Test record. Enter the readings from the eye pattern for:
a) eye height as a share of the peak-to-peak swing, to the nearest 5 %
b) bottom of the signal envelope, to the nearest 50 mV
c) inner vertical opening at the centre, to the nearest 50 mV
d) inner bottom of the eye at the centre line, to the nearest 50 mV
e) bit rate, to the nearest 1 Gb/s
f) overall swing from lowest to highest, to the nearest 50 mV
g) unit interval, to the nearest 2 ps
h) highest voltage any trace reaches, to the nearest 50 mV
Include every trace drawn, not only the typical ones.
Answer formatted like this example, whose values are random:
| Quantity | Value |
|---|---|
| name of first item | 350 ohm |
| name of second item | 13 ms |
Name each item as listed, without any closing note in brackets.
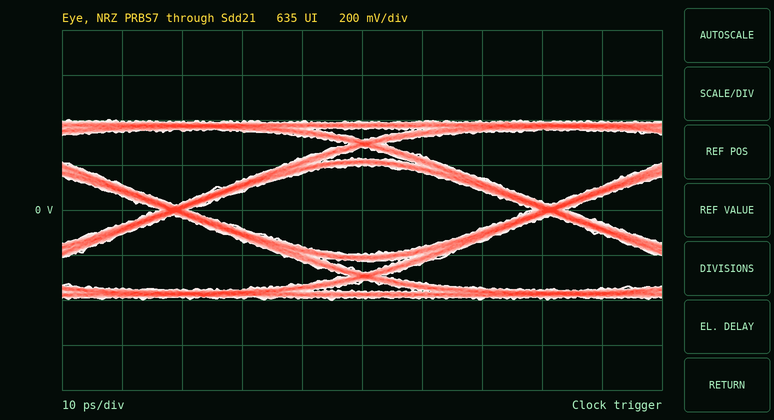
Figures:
| Quantity | Value |
|---|---|
| eye height as a share of the peak-to-peak swing, to the nearest 5 % | 50 % |
| bottom of the signal envelope, to the nearest 50 mV | -400 mV |
| inner vertical opening at the centre, to the nearest 50 mV | 400 mV |
| inner bottom of the eye at the centre line, to the nearest 50 mV | -200 mV |
| bit rate, to the nearest 1 Gb/s | 16 Gb/s |
| overall swing from lowest to highest, to the nearest 50 mV | 800 mV |
| unit interval, to the nearest 2 ps | 62 ps |
| highest voltage any trace reaches, to the nearest 50 mV | 400 mV |
